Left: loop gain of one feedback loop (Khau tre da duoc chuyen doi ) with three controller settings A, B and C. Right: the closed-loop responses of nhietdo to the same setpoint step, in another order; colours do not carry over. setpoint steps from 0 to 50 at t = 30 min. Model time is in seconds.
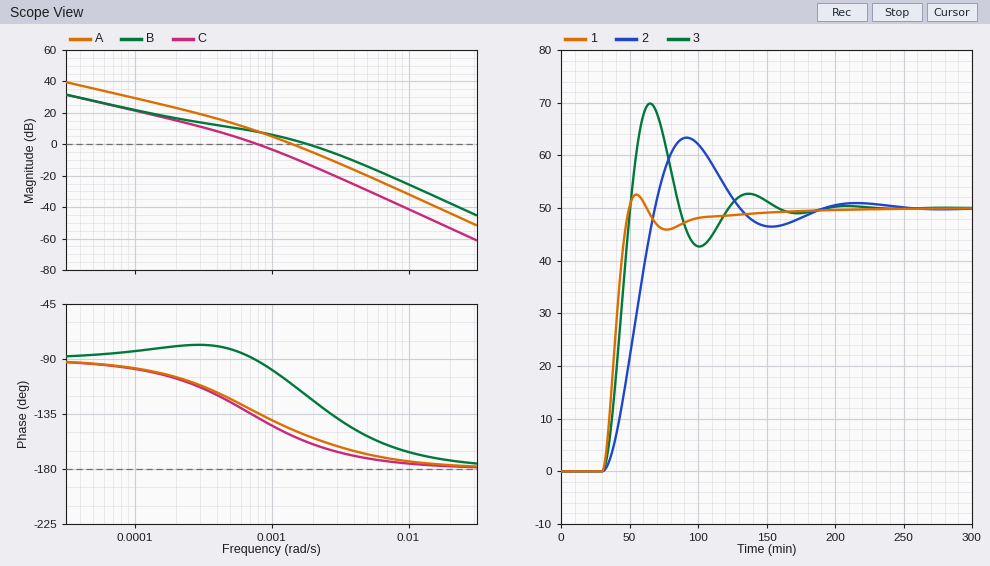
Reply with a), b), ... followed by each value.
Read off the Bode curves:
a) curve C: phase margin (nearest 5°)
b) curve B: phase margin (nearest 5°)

a) 40°
b) 60°
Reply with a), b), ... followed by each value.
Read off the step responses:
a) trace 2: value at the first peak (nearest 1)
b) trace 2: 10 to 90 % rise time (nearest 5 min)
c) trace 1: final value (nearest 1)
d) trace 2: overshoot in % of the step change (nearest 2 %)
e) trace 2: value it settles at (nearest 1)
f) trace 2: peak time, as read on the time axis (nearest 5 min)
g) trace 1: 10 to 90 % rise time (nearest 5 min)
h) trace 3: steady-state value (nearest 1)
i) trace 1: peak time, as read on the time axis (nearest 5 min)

a) 63
b) 25 min
c) 50
d) 26 %
e) 50
f) 90 min
g) 15 min
h) 50
i) 55 min
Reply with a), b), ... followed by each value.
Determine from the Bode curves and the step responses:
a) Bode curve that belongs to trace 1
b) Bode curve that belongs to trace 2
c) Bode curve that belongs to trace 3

a) B
b) C
c) A
